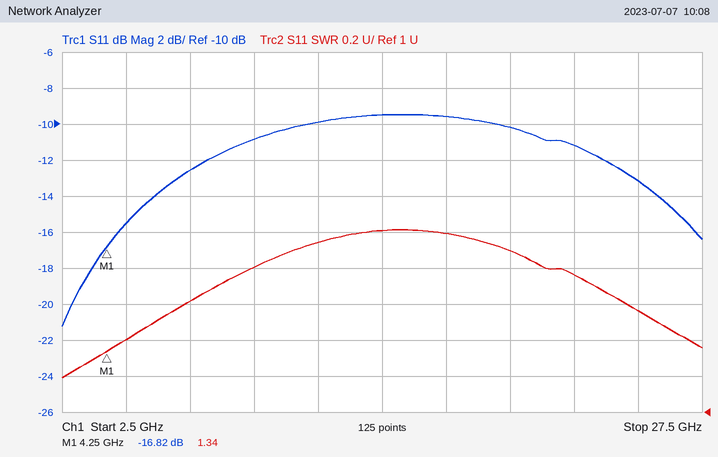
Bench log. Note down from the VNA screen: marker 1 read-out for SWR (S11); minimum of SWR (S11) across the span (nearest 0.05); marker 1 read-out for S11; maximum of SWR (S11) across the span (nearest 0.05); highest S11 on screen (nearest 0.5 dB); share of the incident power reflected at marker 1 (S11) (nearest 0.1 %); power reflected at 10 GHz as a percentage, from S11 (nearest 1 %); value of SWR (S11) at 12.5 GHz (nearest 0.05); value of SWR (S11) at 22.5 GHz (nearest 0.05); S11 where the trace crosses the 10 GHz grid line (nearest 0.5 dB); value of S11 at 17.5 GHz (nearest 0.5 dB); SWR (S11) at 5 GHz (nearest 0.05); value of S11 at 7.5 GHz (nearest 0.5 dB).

1.34
1.20
-16.82 dB
2.00
-9.5 dB
2.1 %
8 %
1.95
1.75
-11.0 dB
-9.5 dB
1.40
-12.5 dB
